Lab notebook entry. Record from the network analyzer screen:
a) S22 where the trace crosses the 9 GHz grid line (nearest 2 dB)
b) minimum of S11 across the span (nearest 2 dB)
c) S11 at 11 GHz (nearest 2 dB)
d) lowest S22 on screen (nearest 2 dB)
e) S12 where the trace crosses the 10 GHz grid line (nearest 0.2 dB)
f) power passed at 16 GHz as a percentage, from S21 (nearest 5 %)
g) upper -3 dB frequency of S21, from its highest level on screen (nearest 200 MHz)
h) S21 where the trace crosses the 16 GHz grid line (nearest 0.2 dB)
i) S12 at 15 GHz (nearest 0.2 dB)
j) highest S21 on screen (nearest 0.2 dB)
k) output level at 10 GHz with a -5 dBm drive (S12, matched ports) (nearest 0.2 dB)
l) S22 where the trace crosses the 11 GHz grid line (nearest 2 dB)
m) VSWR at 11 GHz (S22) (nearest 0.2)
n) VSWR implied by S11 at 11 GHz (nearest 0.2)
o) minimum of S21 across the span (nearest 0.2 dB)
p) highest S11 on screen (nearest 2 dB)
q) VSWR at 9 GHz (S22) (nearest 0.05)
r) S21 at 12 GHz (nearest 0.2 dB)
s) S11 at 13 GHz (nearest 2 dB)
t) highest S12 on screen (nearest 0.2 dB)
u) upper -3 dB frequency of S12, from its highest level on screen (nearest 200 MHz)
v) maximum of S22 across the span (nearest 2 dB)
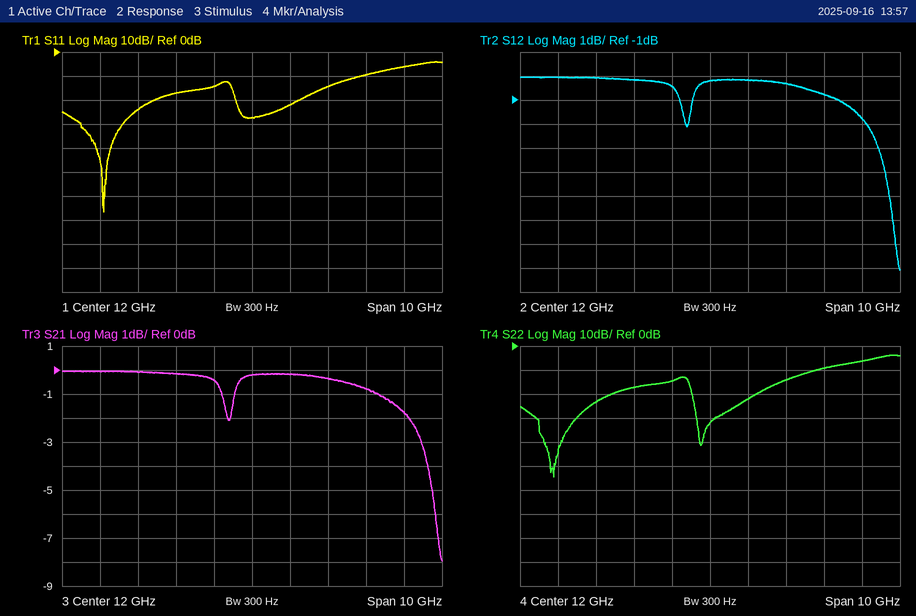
-24 dB
-66 dB
-14 dB
-54 dB
-0.2 dB
65 %
16.4 GHz
-1.8 dB
-0.8 dB
0.0 dB
-5.2 dBm
-14 dB
1.4
1.4
-8.0 dB
-4 dB
1.15
-0.2 dB
-22 dB
0.0 dB
16.4 GHz
-4 dB
